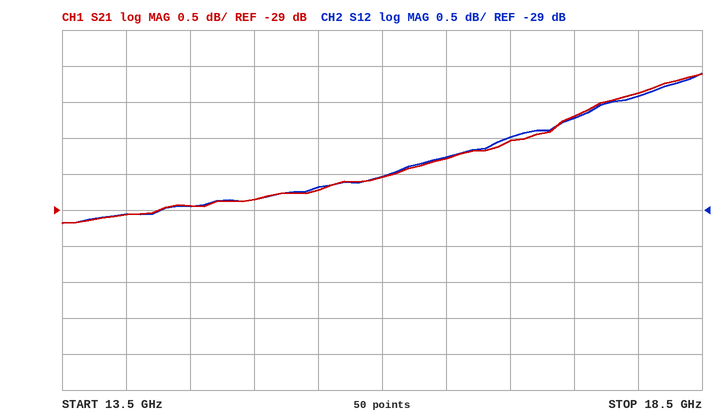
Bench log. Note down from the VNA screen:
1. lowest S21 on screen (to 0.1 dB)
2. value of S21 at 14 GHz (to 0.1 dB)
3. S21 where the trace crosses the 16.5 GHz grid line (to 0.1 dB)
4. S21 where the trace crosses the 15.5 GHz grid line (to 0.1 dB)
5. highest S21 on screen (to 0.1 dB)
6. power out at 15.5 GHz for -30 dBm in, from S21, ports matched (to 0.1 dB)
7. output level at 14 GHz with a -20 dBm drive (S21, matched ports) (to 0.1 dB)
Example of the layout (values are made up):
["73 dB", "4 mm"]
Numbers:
["-29.2 dB", "-29.1 dB", "-28.3 dB", "-28.7 dB", "-27.1 dB", "-58.7 dBm", "-49.1 dBm"]
